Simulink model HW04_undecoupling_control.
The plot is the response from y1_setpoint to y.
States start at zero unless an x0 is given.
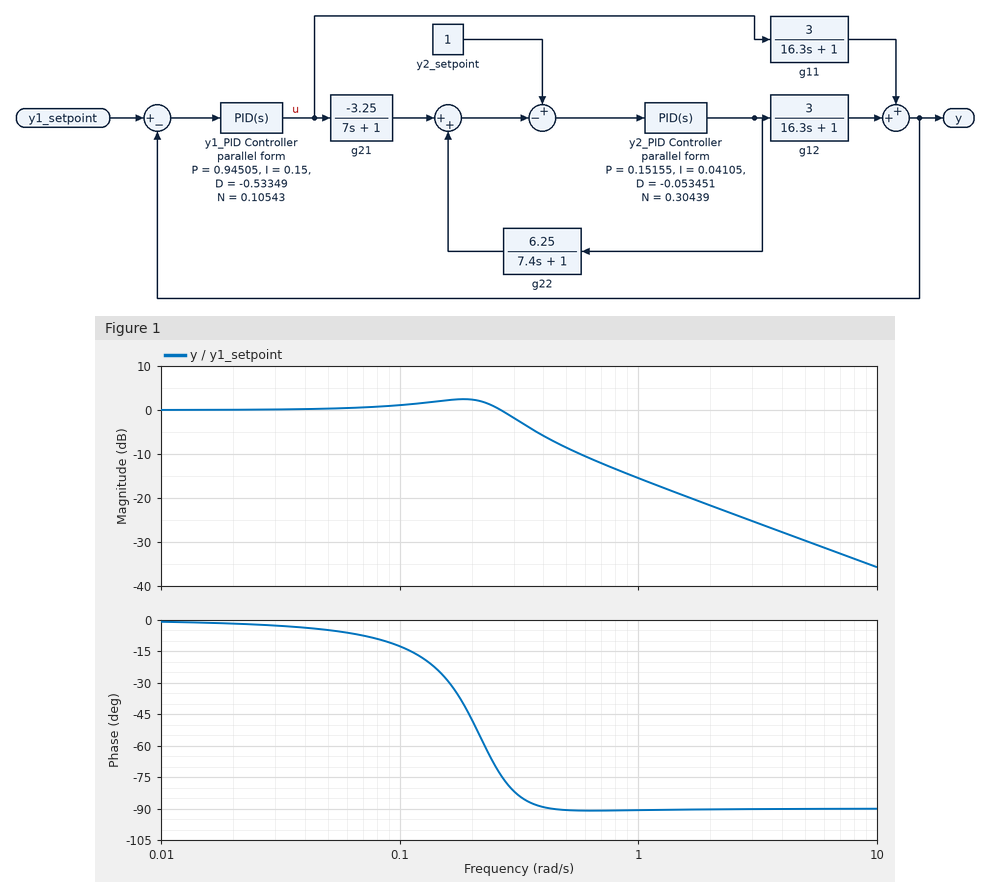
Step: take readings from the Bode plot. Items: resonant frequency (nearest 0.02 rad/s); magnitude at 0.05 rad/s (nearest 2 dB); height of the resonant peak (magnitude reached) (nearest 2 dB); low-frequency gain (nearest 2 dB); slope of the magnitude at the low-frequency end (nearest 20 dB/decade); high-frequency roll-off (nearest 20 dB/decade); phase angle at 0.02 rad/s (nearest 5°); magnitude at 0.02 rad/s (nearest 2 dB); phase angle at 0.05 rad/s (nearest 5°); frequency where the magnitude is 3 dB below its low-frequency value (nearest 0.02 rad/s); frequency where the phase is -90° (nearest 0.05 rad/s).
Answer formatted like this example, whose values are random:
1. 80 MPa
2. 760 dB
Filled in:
1. 0.18 rad/s
2. 0 dB
3. 2 dB
4. 0 dB
5. 0 dB/decade
6. -20 dB/decade
7. 0°
8. 0 dB
9. -5°
10. 0.32 rad/s
11. 0.45 rad/s
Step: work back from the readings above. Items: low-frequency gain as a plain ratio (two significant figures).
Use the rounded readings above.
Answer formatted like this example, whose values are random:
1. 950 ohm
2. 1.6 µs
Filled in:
1. 1.0
